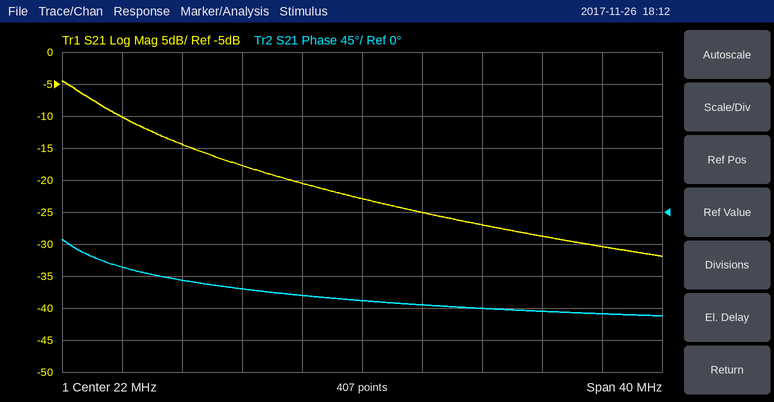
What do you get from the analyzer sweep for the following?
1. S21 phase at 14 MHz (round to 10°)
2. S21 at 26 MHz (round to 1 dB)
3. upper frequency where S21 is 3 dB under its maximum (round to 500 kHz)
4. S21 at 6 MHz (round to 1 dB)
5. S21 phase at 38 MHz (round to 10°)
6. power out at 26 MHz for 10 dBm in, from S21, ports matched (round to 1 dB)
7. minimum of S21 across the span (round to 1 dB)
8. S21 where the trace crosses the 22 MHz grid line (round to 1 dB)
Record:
-110°
-25 dB
4.0 MHz
-10 dB
-140°
-15 dBm
-32 dB
-23 dB
